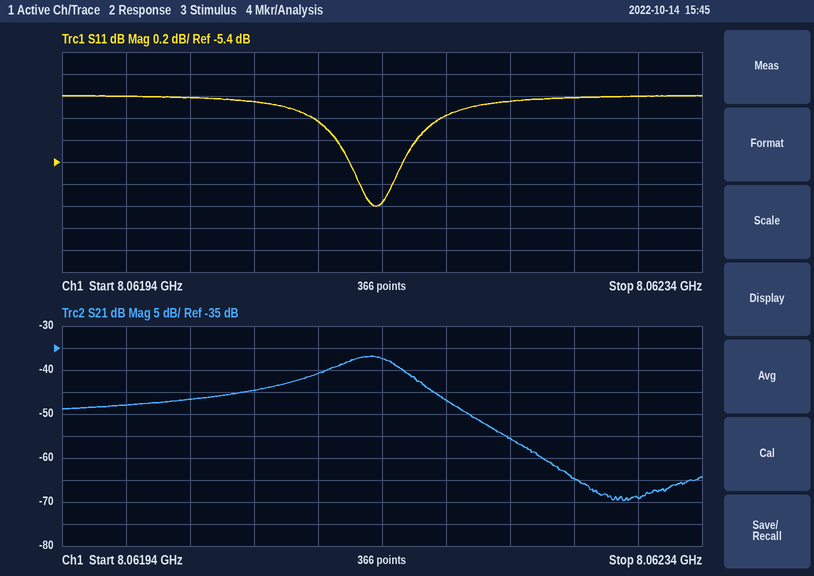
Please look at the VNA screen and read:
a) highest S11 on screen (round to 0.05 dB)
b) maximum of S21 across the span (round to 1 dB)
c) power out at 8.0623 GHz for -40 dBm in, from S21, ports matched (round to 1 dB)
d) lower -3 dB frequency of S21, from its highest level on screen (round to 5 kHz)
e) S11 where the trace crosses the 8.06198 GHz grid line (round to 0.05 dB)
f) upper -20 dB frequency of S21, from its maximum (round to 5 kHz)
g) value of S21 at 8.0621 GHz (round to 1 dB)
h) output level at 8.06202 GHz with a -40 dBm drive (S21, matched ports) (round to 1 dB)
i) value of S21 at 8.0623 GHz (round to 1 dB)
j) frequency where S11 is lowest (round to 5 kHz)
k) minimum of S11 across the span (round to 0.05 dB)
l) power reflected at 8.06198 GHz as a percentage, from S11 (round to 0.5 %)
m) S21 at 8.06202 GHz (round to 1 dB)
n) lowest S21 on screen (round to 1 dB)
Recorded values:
-4.80 dB
-37 dB
-109 dBm
8.062105 GHz
-4.80 dB
8.062225 GHz
-41 dB
-87 dBm
-69 dB
8.062135 GHz
-5.80 dB
33.0 %
-47 dB
-70 dB
